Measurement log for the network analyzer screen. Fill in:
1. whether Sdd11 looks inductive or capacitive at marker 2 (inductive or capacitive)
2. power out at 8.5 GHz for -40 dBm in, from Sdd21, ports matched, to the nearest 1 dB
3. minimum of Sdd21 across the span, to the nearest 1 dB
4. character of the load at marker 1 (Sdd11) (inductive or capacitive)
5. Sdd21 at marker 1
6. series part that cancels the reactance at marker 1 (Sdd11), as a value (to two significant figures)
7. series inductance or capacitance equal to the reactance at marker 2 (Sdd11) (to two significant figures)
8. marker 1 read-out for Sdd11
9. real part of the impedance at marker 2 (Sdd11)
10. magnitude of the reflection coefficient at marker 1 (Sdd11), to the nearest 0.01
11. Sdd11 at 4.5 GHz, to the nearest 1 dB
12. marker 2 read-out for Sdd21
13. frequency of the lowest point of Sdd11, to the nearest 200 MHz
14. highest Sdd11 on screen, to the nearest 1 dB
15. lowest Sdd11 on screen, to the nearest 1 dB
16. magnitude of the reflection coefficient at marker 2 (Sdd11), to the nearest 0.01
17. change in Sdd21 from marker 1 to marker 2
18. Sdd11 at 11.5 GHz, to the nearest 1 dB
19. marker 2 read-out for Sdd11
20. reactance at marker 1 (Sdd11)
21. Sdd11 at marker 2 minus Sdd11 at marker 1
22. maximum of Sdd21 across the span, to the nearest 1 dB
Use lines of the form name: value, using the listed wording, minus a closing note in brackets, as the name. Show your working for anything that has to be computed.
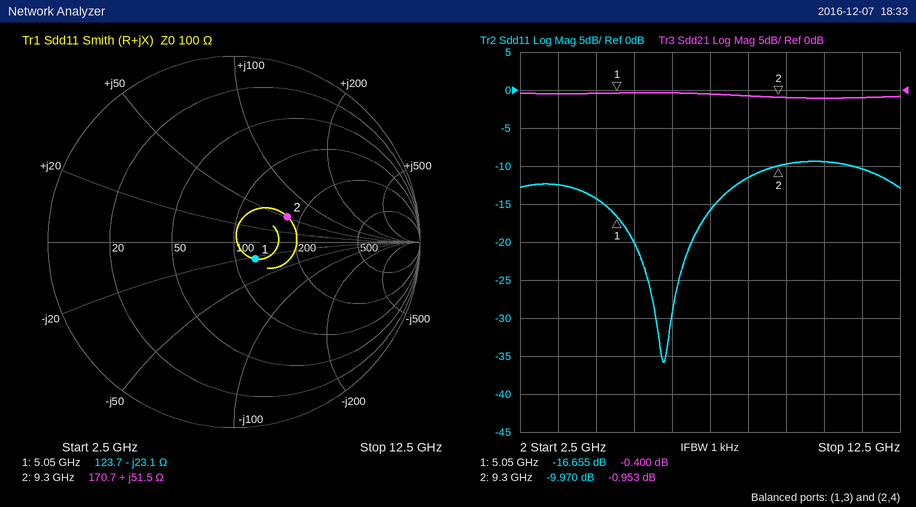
whether Sdd11 looks inductive or capacitive at marker 2: inductive
power out at 8.5 GHz for -40 dBm in, from Sdd21, ports matched, to the nearest 1 dB: -40 dBm + (-1 dB) = -41 dBm
minimum of Sdd21 across the span, to the nearest 1 dB: -1 dB
character of the load at marker 1 (Sdd11): capacitive
Sdd21 at marker 1: -0.400 dB
series part that cancels the reactance at marker 1 (Sdd11), as a value: L = 23.1 Ω/(2π × 5.05 GHz) ≈ 728 pH, so 730 pH to two significant figures
series inductance or capacitance equal to the reactance at marker 2 (Sdd11): L = 51.5 Ω/(2π × 9.3 GHz) ≈ 881 pH, so 880 pH to two significant figures
marker 1 read-out for Sdd11: -16.655 dB
real part of the impedance at marker 2: 170.7 Ω
magnitude of the reflection coefficient at marker 1 (Sdd11), to the nearest 0.01: 0.15
Sdd11 at 4.5 GHz, to the nearest 1 dB: -14 dB
marker 2 read-out for Sdd21: -0.953 dB
frequency of the lowest point of Sdd11, to the nearest 200 MHz: 6.2 GHz
highest Sdd11 on screen, to the nearest 1 dB: -9 dB
lowest Sdd11 on screen, to the nearest 1 dB: -36 dB
magnitude of the reflection coefficient at marker 2 (Sdd11), to the nearest 0.01: 0.32
change in Sdd21 from marker 1 to marker 2: -0.953 − (-0.4) = -0.553 dB
Sdd11 at 11.5 GHz, to the nearest 1 dB: -10 dB
marker 2 read-out for Sdd11: -9.970 dB
reactance at marker 1: -23.1 Ω
Sdd11 at marker 2 minus Sdd11 at marker 1: -9.97 − (-16.655) = 6.685 dB
maximum of Sdd21 across the span, to the nearest 1 dB: 0 dB
